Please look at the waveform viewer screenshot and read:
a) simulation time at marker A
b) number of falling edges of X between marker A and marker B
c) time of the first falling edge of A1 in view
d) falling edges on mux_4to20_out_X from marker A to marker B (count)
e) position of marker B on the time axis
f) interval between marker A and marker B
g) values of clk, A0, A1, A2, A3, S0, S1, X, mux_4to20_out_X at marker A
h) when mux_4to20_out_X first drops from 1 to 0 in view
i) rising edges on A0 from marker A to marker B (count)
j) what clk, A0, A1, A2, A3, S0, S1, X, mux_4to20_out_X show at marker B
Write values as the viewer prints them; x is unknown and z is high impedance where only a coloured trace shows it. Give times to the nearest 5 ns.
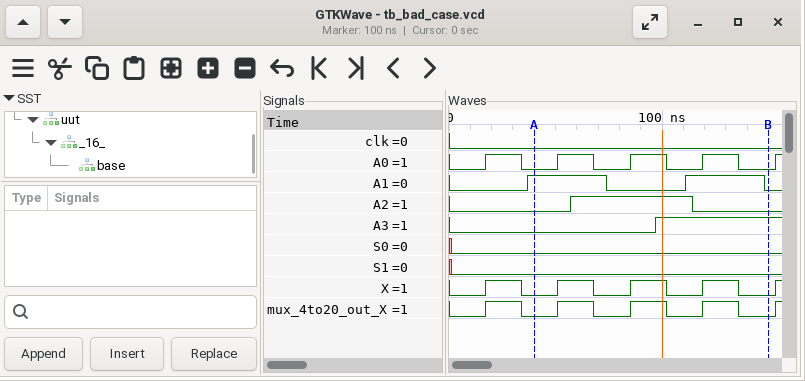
40 ns
3
75 ns
3
150 ns
110 ns
clk=0, A0=0, A1=1, A2=0, A3=0, S0=0, S1=0, X=0, mux_4to20_out_X=0
35 ns
3
clk=0, A0=0, A1=0, A2=0, A3=1, S0=0, S1=0, X=0, mux_4to20_out_X=0
